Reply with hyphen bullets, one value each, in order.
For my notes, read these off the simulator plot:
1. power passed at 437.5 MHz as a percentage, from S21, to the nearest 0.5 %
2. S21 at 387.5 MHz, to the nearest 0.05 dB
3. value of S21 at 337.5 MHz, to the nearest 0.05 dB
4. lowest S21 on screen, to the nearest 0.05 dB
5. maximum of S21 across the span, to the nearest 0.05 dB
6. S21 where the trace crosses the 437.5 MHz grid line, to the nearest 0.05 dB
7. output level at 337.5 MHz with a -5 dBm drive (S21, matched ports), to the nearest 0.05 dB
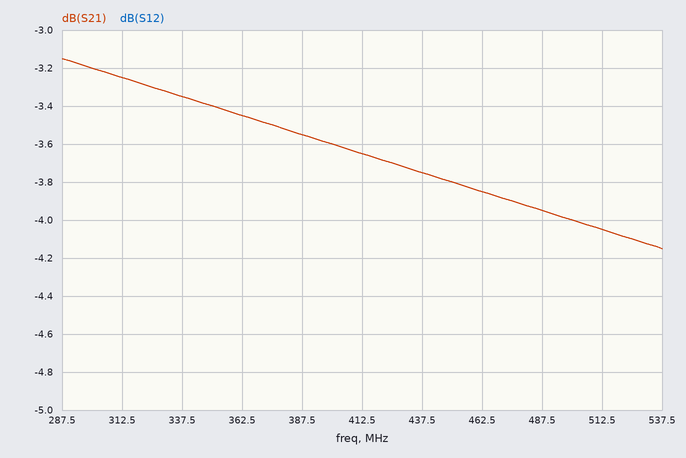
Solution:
- 42.0 %
- -3.55 dB
- -3.35 dB
- -4.15 dB
- -3.15 dB
- -3.75 dB
- -8.35 dBm
